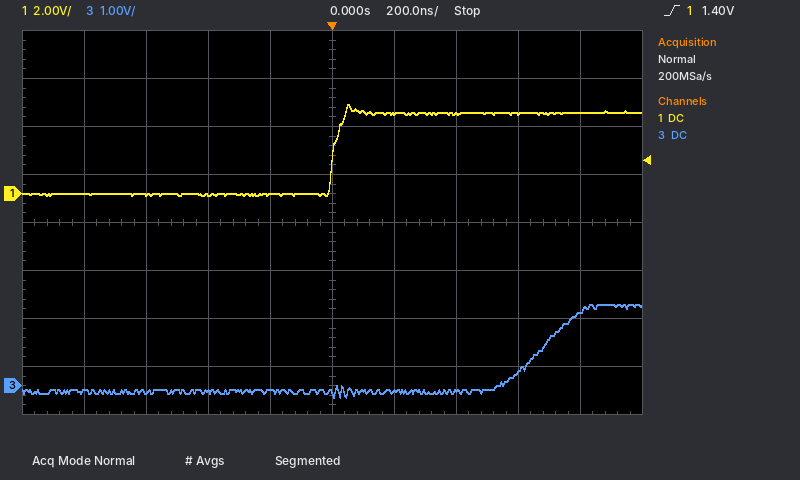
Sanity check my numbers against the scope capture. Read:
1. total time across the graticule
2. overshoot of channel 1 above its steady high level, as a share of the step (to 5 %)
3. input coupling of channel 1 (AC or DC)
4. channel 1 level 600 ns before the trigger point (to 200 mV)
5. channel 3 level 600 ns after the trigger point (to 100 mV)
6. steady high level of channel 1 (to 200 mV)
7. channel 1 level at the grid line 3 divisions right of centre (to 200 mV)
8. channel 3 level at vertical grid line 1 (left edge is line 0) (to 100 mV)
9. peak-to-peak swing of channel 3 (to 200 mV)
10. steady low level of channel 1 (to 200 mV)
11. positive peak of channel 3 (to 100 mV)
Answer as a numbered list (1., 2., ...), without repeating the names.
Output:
1. 2 µs
2. 10 %
3. DC
4. 0.0 V
5. 300 mV
6. 3.4 V
7. 3.4 V
8. -100 mV
9. 2.0 V
10. 0.0 V
11. 1.7 V
